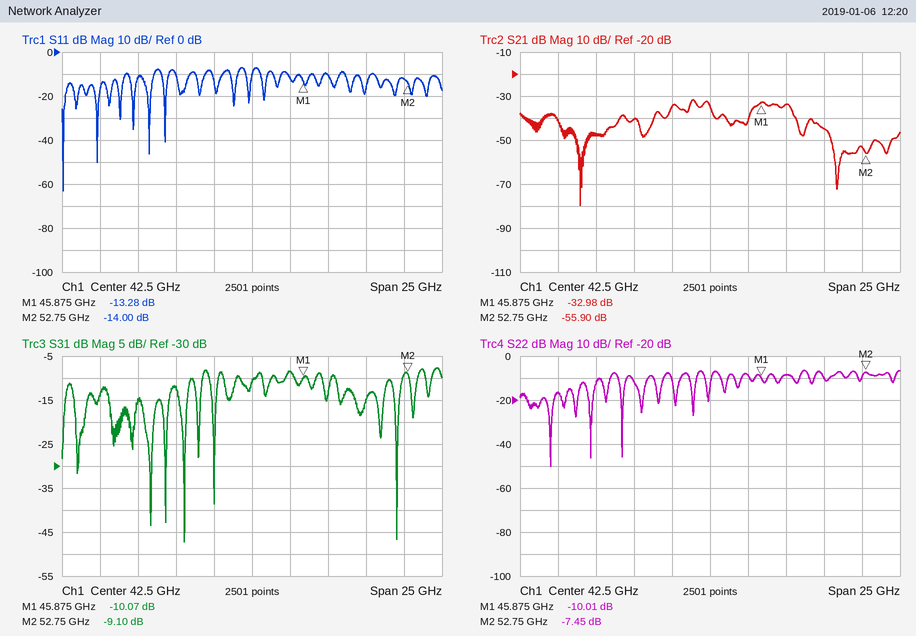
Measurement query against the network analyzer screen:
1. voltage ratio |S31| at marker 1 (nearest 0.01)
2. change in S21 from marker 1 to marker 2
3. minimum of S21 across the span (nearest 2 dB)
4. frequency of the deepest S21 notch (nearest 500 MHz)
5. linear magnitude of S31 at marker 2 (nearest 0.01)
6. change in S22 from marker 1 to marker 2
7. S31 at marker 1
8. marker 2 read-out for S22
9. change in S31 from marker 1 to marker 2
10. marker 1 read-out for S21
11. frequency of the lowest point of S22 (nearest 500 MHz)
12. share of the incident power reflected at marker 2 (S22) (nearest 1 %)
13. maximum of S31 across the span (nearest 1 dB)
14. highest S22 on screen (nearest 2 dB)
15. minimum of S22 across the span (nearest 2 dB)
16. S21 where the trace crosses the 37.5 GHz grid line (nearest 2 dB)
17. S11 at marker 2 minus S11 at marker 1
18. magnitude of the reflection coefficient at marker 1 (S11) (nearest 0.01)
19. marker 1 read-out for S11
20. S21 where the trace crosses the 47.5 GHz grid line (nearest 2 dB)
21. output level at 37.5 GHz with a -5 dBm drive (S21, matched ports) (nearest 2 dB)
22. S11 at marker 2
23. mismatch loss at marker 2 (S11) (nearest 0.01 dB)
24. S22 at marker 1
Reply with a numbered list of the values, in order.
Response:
1. 0.31
2. -22.92 dB
3. -80 dB
4. 34.0 GHz
5. 0.35
6. 2.56 dB
7. -10.07 dB
8. -7.45 dB
9. 0.97 dB
10. -32.98 dB
11. 32.0 GHz
12. 18 %
13. -8 dB
14. -6 dB
15. -50 dB
16. -40 dB
17. -0.72 dB
18. 0.22
19. -13.28 dB
20. -34 dB
21. -46 dBm
22. -14.00 dB
23. 0.18 dB
24. -10.01 dB
